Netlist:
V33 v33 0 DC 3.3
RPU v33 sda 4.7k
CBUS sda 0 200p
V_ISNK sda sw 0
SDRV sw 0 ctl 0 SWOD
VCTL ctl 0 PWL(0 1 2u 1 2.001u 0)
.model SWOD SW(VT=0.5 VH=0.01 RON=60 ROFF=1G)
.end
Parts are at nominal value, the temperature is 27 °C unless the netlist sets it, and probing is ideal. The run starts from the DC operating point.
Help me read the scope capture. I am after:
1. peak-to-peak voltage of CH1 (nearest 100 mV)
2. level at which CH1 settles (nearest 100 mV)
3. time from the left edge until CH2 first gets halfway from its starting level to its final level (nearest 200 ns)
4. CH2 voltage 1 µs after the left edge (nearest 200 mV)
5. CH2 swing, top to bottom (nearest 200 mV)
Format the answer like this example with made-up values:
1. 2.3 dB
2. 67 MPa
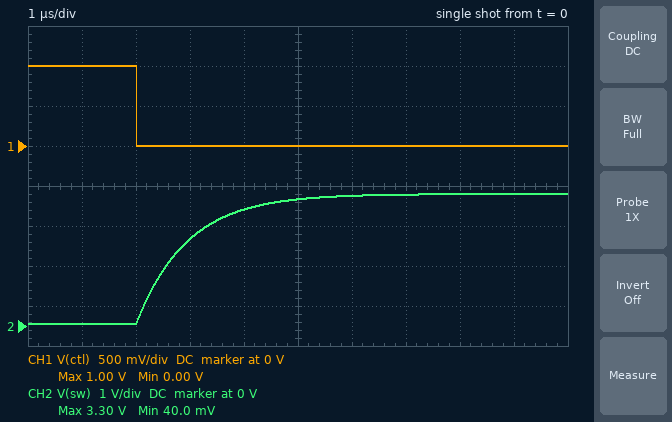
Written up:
1. 1.0 V
2. 0 V
3. 2.6 µs
4. 0 V
5. 3.2 V
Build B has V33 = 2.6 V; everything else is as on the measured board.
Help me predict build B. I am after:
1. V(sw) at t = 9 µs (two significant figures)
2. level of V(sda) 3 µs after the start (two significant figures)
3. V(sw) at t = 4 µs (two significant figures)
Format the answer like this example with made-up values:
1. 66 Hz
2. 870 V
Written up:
1. 2.6 V
2. 1.7 V
3. 2.3 V
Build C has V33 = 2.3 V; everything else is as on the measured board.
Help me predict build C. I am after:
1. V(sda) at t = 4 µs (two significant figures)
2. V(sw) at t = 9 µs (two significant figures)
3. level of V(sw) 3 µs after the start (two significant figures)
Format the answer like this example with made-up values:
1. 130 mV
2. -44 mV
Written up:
1. 2.0 V
2. 2.3 V
3. 1.5 V
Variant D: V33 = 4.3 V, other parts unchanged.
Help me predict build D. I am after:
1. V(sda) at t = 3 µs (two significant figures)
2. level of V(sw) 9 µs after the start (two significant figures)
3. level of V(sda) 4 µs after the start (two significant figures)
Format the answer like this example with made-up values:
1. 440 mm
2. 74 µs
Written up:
1. 2.8 V
2. 4.3 V
3. 3.8 V
